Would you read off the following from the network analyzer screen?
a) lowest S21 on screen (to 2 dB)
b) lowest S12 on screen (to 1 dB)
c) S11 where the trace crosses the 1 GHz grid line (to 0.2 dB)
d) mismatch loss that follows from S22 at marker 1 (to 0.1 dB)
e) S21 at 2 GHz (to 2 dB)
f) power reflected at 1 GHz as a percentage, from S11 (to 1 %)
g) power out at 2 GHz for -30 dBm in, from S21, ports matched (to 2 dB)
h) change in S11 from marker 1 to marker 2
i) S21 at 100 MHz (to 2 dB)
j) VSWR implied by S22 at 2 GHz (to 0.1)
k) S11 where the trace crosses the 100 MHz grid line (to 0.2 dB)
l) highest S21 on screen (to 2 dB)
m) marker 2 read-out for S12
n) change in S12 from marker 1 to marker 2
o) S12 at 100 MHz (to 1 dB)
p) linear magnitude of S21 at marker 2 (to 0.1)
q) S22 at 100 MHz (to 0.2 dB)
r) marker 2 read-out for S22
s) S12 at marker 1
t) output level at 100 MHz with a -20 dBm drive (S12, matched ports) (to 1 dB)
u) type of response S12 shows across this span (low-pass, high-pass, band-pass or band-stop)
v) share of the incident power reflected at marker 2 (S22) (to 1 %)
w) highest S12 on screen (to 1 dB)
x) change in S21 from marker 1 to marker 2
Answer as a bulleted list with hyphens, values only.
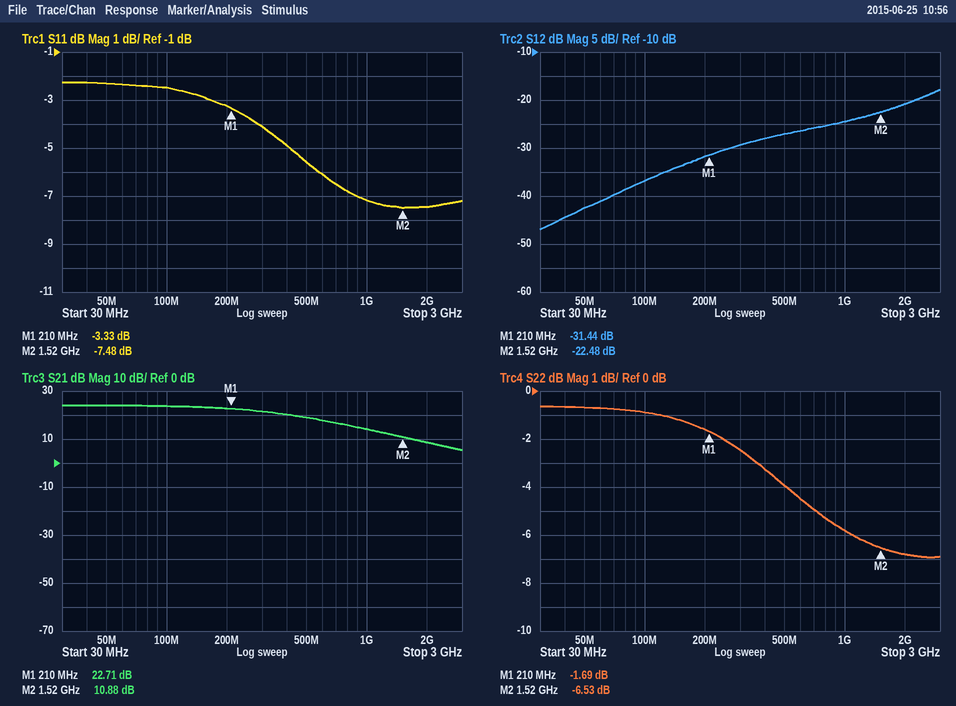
- 6 dB
- -47 dB
- -7.2 dB
- 4.9 dB
- 8 dB
- 19 %
- -22 dBm
- -4.15 dB
- 24 dB
- 2.7
- -2.4 dB
- 24 dB
- -22.48 dB
- 8.96 dB
- -37 dB
- 3.5
- -0.8 dB
- -6.53 dB
- -31.44 dB
- -57 dBm
- high-pass
- 22 %
- -18 dB
- -11.83 dB
